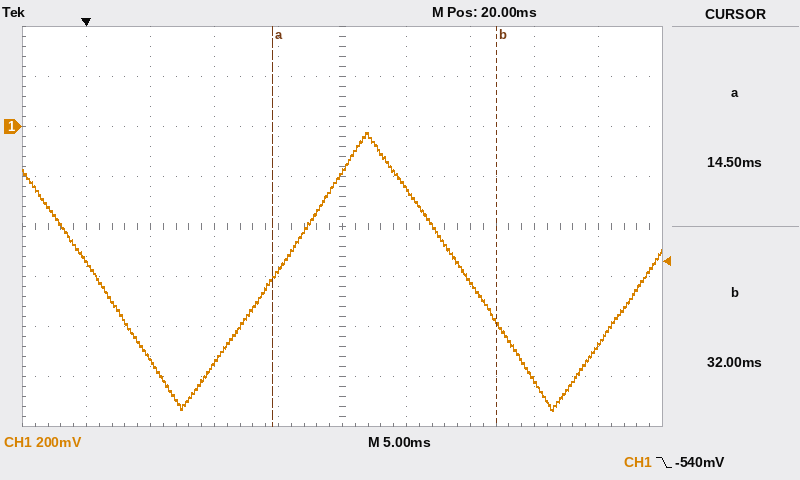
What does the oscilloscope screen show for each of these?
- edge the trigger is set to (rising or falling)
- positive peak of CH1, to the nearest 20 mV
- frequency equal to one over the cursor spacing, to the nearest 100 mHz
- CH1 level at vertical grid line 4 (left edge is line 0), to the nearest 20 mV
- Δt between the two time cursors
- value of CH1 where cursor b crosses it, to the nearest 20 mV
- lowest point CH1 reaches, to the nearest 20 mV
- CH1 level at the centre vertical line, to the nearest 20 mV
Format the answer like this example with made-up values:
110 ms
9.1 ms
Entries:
falling
-20 mV
57.1 Hz
-580 mV
17.5 ms
-780 mV
-1.14 V
-180 mV
